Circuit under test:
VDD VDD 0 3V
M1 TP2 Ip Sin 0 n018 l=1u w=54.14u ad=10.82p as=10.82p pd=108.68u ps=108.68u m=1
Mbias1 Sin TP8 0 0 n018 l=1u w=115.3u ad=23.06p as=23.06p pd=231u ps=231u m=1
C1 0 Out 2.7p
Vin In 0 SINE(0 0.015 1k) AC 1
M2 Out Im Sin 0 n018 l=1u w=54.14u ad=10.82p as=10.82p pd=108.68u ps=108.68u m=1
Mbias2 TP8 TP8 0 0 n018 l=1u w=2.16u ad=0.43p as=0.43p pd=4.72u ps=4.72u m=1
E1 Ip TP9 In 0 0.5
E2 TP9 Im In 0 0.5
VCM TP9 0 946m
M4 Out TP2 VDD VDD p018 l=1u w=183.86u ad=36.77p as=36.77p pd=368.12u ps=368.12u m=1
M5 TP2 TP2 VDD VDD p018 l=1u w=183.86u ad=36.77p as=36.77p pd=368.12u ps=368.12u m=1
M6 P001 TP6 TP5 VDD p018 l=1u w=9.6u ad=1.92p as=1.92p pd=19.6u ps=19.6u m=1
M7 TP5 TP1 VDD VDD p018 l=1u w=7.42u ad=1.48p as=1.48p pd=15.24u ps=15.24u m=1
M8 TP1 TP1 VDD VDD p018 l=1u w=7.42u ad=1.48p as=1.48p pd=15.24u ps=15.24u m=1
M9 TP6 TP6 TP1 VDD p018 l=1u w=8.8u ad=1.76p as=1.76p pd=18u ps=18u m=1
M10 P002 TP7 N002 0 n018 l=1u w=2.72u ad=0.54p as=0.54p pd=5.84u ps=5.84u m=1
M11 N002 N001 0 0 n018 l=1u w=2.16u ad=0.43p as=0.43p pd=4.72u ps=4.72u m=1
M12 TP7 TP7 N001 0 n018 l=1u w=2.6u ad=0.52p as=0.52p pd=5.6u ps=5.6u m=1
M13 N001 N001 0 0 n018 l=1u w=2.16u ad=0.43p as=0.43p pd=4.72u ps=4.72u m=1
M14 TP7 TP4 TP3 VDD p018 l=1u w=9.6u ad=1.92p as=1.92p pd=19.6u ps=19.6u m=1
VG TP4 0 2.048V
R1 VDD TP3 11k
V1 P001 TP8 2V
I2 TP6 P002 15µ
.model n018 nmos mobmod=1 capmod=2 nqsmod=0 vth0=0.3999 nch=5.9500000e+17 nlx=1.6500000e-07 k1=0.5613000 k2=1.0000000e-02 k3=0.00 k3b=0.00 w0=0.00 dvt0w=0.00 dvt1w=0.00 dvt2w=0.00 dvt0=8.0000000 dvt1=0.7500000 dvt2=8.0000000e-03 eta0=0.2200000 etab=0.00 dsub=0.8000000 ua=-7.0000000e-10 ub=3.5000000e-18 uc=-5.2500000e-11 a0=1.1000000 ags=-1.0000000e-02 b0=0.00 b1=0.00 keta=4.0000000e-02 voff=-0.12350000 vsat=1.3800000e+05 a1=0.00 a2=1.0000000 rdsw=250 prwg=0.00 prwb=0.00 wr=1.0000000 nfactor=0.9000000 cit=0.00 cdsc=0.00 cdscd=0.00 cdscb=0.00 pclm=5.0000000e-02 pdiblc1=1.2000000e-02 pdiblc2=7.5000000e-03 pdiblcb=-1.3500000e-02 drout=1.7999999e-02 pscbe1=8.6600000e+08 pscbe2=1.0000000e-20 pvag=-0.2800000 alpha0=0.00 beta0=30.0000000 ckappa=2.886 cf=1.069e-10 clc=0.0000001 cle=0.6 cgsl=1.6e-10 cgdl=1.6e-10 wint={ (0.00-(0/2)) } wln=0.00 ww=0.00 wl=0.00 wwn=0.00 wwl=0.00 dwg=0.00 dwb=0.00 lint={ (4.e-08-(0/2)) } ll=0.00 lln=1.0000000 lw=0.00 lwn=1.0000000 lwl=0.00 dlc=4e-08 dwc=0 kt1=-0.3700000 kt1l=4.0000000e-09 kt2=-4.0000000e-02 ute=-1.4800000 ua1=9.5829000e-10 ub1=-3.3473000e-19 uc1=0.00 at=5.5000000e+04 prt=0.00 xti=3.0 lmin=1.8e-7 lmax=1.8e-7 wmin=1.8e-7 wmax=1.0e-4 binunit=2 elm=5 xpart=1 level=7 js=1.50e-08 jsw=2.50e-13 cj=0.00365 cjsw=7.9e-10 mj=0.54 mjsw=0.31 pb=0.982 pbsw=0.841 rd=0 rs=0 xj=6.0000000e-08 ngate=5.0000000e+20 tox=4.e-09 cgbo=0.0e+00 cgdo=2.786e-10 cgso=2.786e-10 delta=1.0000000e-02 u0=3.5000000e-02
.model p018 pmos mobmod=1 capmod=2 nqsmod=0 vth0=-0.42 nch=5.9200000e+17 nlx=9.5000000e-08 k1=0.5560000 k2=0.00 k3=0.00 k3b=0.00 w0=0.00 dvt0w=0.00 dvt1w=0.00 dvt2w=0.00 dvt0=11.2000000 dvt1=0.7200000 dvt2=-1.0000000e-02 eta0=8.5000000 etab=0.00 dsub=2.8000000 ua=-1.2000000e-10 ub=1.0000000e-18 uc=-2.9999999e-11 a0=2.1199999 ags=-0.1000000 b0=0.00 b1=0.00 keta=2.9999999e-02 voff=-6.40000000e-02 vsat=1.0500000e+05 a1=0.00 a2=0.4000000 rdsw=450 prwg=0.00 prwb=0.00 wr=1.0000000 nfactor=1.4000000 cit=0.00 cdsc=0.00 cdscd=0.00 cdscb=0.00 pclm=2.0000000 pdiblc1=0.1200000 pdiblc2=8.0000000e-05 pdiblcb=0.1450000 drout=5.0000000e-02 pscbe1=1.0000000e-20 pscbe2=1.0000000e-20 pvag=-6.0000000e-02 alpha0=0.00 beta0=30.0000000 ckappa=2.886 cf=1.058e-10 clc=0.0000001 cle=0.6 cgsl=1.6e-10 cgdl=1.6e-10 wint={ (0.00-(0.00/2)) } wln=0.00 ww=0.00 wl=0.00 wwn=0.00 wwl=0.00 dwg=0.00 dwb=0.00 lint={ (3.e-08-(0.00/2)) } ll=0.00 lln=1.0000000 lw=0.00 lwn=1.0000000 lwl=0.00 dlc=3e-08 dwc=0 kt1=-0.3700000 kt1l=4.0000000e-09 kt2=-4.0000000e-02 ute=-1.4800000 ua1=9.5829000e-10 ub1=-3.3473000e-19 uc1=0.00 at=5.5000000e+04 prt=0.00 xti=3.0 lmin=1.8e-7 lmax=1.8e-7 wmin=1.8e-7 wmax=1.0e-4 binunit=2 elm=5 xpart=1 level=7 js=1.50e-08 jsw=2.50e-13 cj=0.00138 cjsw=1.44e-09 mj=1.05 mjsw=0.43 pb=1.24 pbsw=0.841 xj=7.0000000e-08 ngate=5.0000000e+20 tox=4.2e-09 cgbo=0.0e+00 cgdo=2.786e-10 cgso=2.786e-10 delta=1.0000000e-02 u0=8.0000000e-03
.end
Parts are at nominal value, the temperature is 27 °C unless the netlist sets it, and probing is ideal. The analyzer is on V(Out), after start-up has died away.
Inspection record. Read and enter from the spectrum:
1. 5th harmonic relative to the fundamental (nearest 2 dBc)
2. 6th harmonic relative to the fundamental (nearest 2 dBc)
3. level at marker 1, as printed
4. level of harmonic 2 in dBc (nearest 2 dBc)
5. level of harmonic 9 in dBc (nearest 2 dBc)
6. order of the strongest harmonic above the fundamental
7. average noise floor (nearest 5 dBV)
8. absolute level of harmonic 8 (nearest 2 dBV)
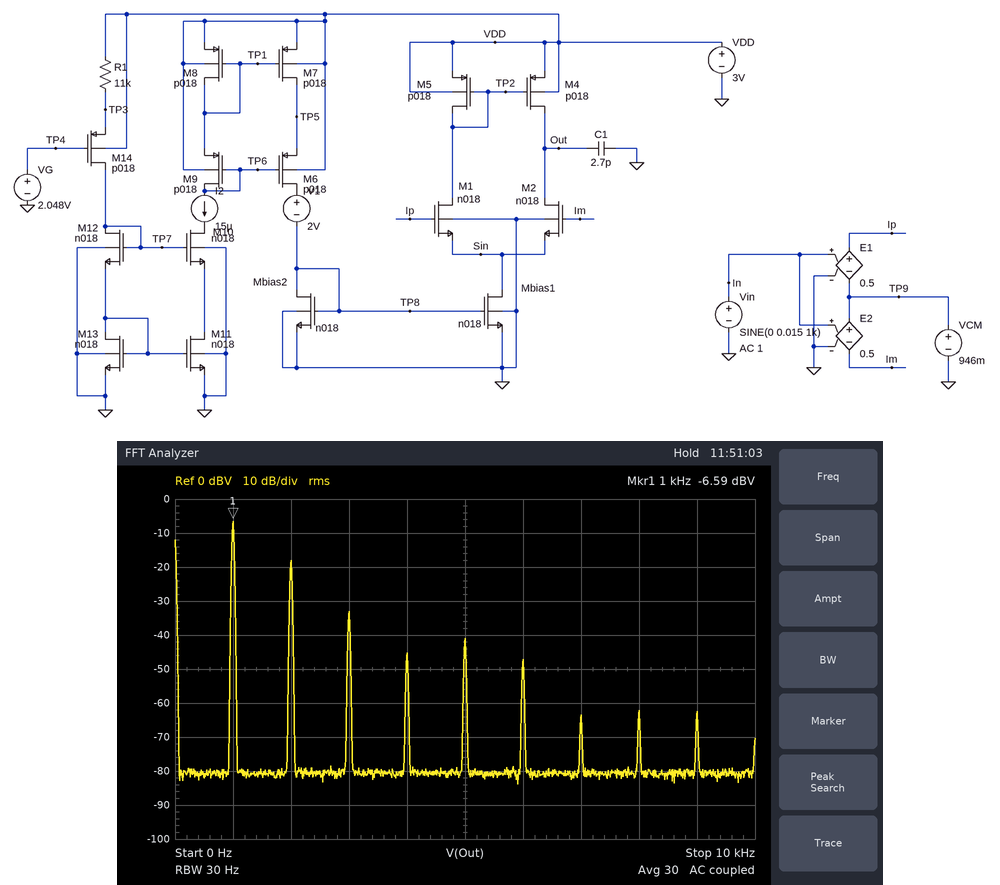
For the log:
-34 dBc
-40 dBc
-6.59 dBV
-12 dBc
-56 dBc
2
-80 dBV
-62 dBV
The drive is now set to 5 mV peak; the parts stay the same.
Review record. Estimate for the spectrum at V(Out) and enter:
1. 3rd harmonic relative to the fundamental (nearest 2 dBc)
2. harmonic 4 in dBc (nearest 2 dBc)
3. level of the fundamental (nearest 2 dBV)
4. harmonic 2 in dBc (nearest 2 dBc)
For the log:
-38 dBc
-56 dBc
-18 dBV
-20 dBc
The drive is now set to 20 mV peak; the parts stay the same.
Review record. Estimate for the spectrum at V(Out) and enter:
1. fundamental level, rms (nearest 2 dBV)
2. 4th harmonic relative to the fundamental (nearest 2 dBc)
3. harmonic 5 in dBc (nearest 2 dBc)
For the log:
-4 dBV
-26 dBc
-30 dBc
